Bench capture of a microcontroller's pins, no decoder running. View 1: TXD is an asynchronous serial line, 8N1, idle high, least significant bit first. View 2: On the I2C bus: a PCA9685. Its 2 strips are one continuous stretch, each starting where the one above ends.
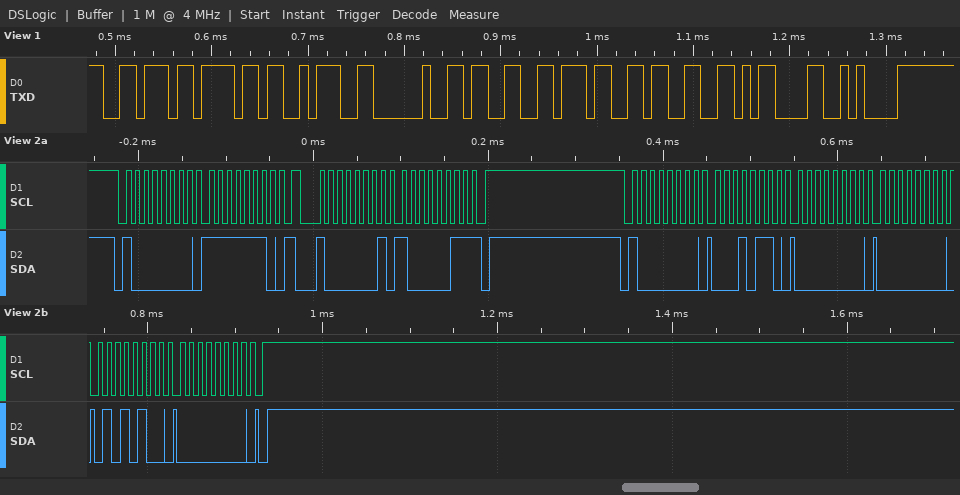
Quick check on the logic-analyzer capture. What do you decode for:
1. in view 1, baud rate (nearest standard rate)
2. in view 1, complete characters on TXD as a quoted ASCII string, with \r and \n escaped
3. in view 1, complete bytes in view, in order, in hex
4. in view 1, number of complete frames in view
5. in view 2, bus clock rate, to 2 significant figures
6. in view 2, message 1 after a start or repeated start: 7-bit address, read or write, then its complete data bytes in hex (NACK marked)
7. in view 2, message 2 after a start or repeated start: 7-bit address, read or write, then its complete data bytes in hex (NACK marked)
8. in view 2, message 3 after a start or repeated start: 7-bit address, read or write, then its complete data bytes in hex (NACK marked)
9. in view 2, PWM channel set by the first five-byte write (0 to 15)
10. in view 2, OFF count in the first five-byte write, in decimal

115200 baud
"vo: 373\r\n"
0x76 0x6F 0x3A 0x20 0x33 0x37 0x33 0x0D 0x0A
9
100 kHz
0x40 write: FE
0x40 read: 83 NACK
0x40 write: 16 00 00 54 00
4
84
